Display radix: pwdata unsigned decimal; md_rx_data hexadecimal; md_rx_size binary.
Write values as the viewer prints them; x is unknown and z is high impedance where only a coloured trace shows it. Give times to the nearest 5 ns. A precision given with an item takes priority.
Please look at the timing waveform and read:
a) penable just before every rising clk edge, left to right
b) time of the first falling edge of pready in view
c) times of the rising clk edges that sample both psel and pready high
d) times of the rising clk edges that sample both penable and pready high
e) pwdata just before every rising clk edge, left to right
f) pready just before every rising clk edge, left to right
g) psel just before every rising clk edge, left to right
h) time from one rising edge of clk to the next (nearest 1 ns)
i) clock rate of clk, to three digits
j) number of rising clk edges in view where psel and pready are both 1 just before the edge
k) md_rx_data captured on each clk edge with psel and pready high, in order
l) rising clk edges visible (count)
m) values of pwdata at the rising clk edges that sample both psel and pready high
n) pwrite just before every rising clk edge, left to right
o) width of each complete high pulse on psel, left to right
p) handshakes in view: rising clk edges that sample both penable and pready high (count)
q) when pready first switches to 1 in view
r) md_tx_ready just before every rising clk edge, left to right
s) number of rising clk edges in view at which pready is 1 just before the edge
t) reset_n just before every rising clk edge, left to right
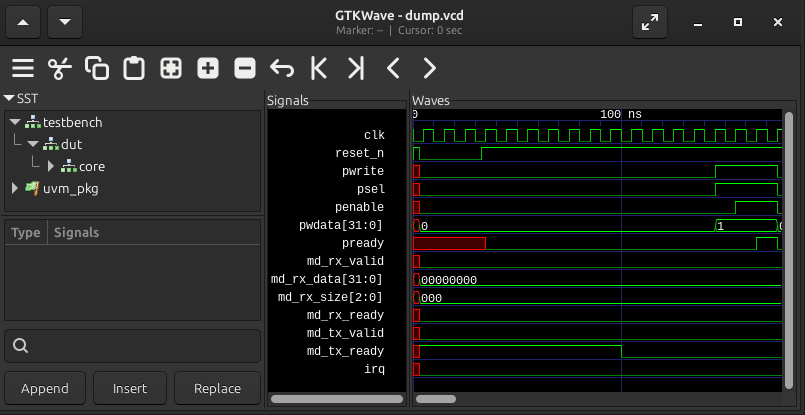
0 0 0 0 0 0 0 0 0 0 0 0 0 0 0 0 1 1
175 ns
175 ns
175 ns
0, 0, 0, 0, 0, 0, 0, 0, 0, 0, 0, 0, 0, 0, 0, 1, 1, 1
x x x x 0 0 0 0 0 0 0 0 0 0 0 0 0 1
0 0 0 0 0 0 0 0 0 0 0 0 0 0 0 1 1 1
10 ns
100 MHz
1
00000000
18
1
0 0 0 0 0 0 0 0 0 0 0 0 0 0 0 1 1 1
30 ns
1
165 ns
1 1 1 1 1 1 1 1 1 1 0 0 0 0 0 0 0 0
1
0 0 0 1 1 1 1 1 1 1 1 1 1 1 1 1 1 1
